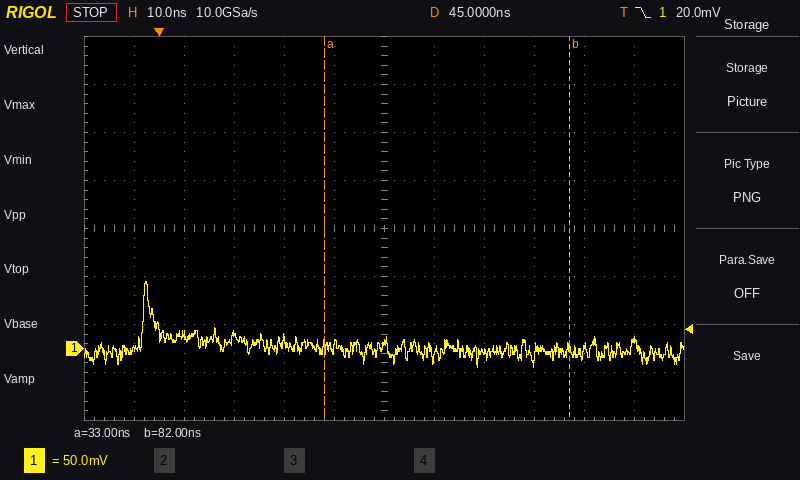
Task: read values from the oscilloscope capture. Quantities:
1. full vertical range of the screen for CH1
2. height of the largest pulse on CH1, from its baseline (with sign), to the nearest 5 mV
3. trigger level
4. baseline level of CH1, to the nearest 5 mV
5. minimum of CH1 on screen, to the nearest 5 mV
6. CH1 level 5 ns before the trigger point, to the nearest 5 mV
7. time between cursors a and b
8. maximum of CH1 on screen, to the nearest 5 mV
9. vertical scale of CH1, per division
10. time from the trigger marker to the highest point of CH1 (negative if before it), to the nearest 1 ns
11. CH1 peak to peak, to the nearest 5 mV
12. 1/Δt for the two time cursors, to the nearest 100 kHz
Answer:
400 mV
+70 mV
20.0 mV
0 mV
-20 mV
0 mV
49 ns
70 mV
50 mV
-3 ns
90 mV
20.4 MHz
